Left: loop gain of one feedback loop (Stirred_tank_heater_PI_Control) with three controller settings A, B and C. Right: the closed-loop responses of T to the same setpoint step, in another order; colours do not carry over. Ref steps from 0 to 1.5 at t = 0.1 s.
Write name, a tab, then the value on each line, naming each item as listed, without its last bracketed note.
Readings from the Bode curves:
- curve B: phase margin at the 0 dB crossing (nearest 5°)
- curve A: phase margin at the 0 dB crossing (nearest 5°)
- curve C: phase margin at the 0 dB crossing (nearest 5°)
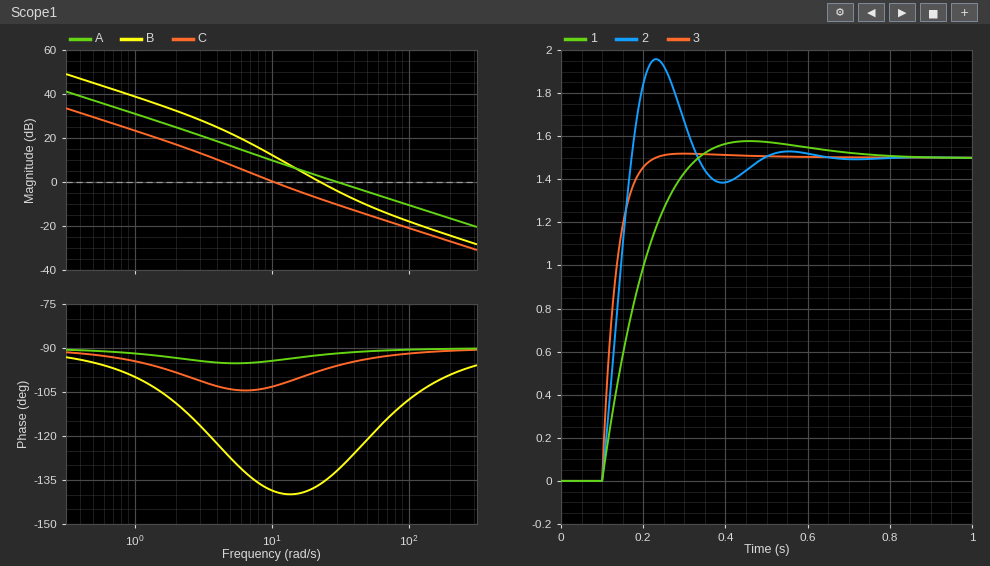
curve B: phase margin at the 0 dB crossing	45°
curve A: phase margin at the 0 dB crossing	90°
curve C: phase margin at the 0 dB crossing	75°
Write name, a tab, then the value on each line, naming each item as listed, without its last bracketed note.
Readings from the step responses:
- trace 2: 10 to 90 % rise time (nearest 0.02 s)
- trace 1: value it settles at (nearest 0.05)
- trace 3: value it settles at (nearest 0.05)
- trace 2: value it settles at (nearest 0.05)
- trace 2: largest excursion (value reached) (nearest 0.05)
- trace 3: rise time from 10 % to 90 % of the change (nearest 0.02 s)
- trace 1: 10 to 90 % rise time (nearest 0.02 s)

trace 2: 10 to 90 % rise time	0.06 s
trace 1: value it settles at	1.50
trace 3: value it settles at	1.50
trace 2: value it settles at	1.50
trace 2: largest excursion (value reached)	1.95
trace 3: rise time from 10 % to 90 % of the change	0.06 s
trace 1: 10 to 90 % rise time	0.16 s
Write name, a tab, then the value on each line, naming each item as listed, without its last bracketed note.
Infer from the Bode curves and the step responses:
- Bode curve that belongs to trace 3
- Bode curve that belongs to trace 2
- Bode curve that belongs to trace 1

Bode curve that belongs to trace 3	A
Bode curve that belongs to trace 2	B
Bode curve that belongs to trace 1	C
